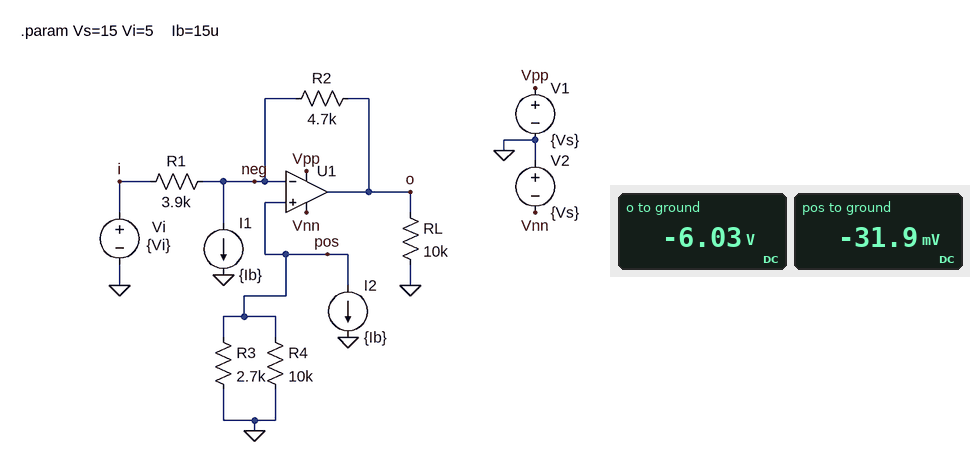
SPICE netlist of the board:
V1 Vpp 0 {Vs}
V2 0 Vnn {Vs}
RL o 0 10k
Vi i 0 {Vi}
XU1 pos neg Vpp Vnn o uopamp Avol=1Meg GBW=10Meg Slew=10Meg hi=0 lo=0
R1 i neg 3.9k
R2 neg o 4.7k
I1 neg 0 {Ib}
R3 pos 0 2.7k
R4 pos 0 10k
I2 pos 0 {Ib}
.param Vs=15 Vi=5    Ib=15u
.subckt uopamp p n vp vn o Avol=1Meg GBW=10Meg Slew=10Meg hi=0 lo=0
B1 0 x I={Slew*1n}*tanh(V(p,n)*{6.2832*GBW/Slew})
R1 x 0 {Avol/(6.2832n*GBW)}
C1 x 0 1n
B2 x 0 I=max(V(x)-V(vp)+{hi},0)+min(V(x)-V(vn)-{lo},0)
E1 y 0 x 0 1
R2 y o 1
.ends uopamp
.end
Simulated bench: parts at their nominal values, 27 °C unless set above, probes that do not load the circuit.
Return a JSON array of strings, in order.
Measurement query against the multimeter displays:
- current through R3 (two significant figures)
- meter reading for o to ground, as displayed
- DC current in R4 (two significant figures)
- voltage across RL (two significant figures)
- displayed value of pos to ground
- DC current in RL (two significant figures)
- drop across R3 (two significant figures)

["12 µA", "-6.03 V", "3.2 µA", "6.0 V", "-31.9 mV", "600 µA", "32 mV"]
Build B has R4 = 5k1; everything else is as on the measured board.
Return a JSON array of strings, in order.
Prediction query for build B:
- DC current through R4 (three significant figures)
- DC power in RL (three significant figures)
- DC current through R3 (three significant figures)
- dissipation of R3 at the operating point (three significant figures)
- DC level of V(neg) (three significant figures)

["5.19 µA", "3.62 mW", "9.81 µA", "260 nW", "-26.5 mV"]
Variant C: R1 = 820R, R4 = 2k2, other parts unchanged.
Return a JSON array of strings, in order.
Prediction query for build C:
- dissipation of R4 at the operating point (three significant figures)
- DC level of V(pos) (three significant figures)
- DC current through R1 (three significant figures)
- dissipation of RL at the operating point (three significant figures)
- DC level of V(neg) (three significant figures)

["150 nW", "-18.2 mV", "3.64 mA", "22.5 mW", "2.02 V"]
